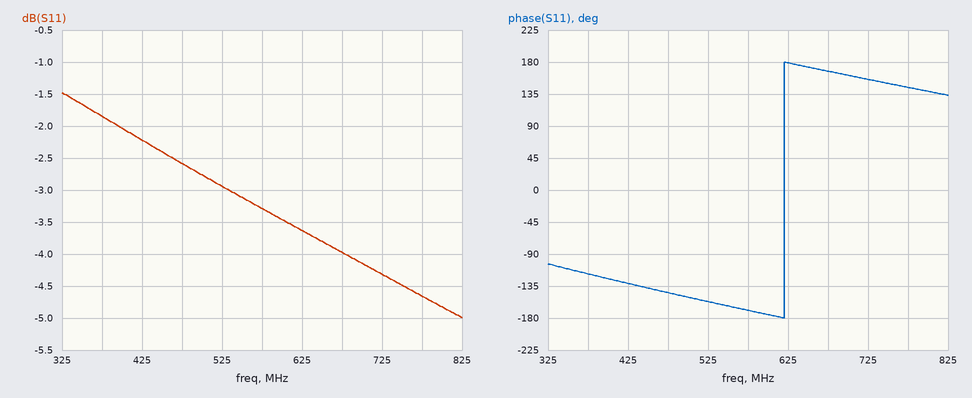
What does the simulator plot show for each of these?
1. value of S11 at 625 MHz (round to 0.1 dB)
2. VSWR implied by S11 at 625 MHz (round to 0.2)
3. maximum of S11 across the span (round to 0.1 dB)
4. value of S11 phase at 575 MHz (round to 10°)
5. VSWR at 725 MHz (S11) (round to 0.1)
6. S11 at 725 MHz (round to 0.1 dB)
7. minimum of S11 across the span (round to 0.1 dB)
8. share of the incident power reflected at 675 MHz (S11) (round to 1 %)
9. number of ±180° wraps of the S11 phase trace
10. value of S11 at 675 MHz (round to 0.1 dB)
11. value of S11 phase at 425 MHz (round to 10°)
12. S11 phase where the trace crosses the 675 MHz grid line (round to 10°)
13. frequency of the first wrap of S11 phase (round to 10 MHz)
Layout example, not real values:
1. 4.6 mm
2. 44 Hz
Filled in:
1. -3.6 dB
2. 4.8
3. -1.5 dB
4. -170°
5. 4.1
6. -4.3 dB
7. -5.0 dB
8. 40 %
9. 1
10. -4.0 dB
11. -130°
12. 170°
13. 620 MHz
